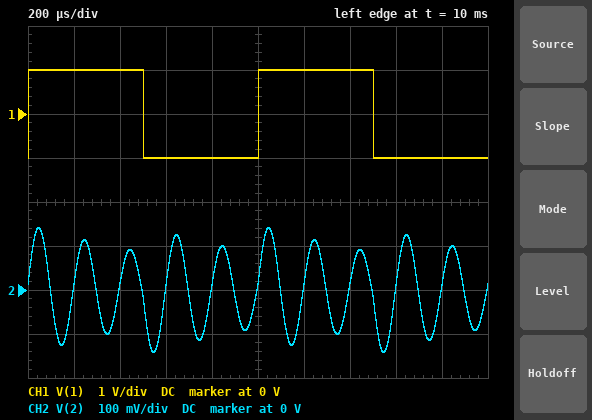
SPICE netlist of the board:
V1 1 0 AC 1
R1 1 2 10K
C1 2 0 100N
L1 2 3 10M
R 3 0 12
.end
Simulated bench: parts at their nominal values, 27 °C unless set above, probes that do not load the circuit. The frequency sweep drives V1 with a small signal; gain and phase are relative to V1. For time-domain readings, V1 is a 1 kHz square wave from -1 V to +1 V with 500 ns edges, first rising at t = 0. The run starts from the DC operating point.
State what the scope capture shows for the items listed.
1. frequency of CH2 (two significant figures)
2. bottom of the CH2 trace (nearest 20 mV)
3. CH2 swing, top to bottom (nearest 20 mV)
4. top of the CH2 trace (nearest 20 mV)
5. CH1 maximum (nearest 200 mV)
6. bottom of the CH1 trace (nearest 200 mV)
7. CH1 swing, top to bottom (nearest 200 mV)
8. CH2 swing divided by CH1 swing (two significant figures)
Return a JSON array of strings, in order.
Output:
["5.0 kHz", "-140 mV", "280 mV", "140 mV", "1.0 V", "-1.0 V", "2.0 V", "0.14"]
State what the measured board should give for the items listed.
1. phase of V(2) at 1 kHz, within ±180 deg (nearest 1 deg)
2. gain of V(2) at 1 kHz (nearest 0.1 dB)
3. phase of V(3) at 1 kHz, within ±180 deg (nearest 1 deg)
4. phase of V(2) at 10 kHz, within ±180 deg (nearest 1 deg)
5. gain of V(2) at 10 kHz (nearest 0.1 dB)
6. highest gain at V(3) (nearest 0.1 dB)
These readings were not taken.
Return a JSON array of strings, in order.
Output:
["78 deg", "-43.5 dB", "-1 deg", "-88 deg", "-33.4 dB", "-35.3 dB"]
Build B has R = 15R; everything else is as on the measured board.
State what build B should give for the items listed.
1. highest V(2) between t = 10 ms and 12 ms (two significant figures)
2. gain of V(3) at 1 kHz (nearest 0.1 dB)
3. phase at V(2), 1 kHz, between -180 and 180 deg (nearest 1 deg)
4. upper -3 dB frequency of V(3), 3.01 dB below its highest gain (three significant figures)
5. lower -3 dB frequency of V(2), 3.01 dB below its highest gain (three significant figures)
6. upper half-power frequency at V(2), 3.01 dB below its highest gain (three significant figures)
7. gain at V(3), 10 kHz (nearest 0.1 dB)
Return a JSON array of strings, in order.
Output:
["130 mV", "-56.1 dB", "76 deg", "5.22 kHz", "4.84 kHz", "5.24 kHz", "-65.9 dB"]
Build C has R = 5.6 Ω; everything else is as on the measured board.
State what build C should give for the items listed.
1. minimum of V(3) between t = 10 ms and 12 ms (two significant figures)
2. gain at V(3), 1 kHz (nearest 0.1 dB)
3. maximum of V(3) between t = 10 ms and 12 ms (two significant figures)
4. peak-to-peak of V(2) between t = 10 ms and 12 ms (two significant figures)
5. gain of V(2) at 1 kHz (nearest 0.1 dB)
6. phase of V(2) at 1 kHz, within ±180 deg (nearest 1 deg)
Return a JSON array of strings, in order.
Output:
["-3.7 mV", "-64.7 dB", "3.7 mV", "370 mV", "-43.7 dB", "84 deg"]
